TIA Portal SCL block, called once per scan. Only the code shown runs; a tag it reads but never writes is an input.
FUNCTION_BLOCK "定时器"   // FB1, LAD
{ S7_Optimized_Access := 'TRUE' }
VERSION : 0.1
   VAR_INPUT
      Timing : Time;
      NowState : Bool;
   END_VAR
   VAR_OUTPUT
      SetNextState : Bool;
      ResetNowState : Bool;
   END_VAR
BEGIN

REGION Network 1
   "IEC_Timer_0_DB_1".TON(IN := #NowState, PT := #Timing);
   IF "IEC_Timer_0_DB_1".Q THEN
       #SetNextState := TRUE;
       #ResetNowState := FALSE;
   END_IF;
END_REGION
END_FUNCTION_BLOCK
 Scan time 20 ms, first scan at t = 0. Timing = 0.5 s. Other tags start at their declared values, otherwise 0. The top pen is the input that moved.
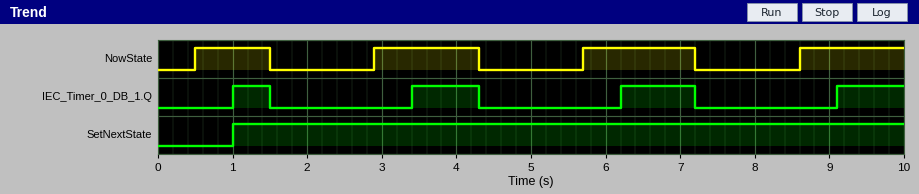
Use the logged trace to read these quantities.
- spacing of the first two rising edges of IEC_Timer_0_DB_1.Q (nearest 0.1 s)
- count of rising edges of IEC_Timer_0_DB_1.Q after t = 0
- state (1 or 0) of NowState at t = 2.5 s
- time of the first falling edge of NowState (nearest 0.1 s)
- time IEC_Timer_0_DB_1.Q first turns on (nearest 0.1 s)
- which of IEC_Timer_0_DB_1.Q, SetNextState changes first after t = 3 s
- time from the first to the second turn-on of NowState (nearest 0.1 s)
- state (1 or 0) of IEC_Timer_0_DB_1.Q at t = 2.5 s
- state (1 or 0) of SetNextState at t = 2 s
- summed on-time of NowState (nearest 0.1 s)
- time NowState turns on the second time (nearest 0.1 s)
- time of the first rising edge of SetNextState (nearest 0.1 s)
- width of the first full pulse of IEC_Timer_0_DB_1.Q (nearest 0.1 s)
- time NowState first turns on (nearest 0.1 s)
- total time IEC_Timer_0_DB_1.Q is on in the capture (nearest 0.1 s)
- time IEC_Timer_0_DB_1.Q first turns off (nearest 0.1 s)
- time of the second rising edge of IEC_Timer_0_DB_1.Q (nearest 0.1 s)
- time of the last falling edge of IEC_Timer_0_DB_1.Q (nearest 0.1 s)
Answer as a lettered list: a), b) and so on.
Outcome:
a) 2.4 s
b) 4
c) 0
d) 1.5 s
e) 1.0 s
f) IEC_Timer_0_DB_1.Q
g) 2.4 s
h) 0
i) 1
j) 5.3 s
k) 2.9 s
l) 1.0 s
m) 0.5 s
n) 0.5 s
o) 3.3 s
p) 1.5 s
q) 3.4 s
r) 7.2 s
